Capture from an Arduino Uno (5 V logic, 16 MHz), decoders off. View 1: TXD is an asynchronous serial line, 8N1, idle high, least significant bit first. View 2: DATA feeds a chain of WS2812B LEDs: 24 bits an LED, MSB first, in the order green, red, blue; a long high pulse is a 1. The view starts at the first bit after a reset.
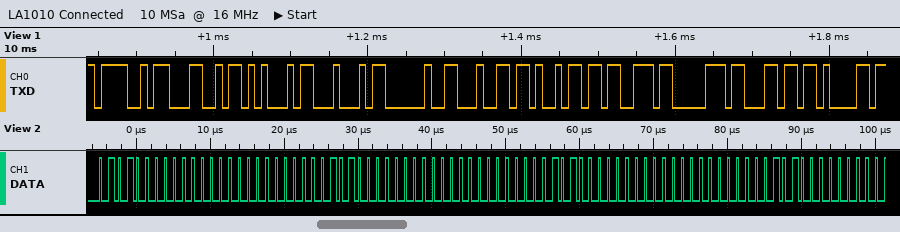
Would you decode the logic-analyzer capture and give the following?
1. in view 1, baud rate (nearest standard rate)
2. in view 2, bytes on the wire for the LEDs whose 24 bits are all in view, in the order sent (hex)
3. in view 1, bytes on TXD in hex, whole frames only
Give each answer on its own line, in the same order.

115200 baud
50 00 00 50 00 00 50 00 00
0x4F 0x4C 0x45 0x44 0x20 0x64 0x69 0x73 0x70 0x6C 0x61
